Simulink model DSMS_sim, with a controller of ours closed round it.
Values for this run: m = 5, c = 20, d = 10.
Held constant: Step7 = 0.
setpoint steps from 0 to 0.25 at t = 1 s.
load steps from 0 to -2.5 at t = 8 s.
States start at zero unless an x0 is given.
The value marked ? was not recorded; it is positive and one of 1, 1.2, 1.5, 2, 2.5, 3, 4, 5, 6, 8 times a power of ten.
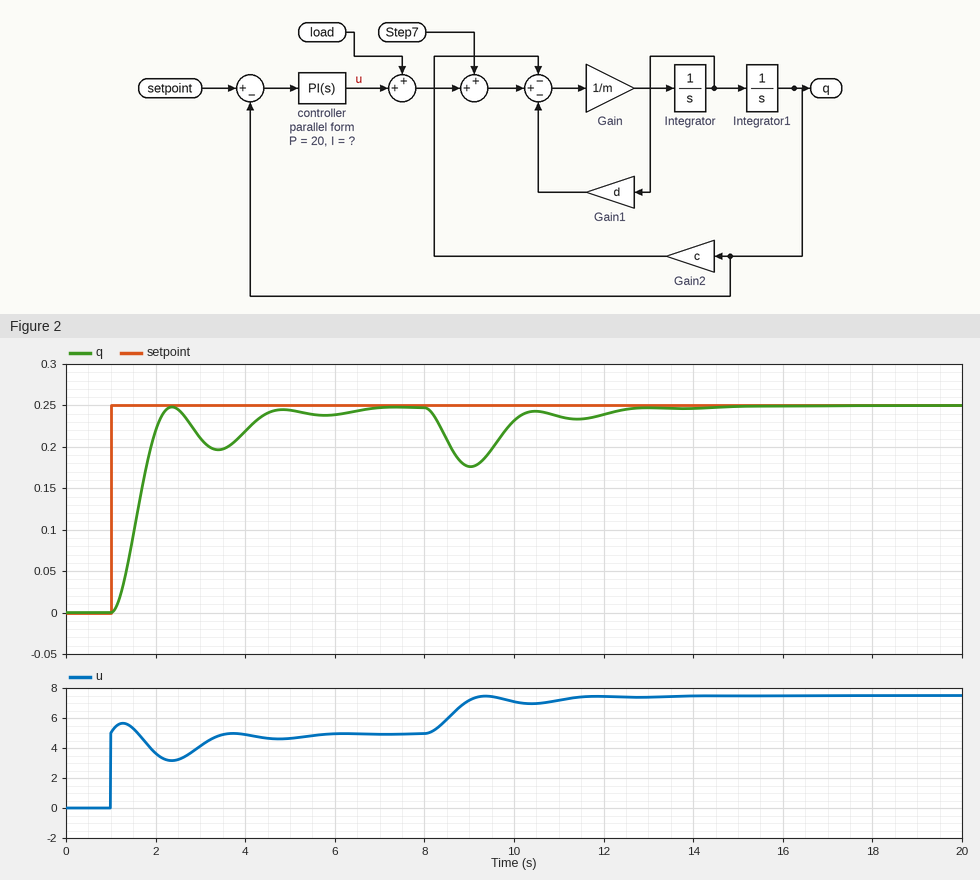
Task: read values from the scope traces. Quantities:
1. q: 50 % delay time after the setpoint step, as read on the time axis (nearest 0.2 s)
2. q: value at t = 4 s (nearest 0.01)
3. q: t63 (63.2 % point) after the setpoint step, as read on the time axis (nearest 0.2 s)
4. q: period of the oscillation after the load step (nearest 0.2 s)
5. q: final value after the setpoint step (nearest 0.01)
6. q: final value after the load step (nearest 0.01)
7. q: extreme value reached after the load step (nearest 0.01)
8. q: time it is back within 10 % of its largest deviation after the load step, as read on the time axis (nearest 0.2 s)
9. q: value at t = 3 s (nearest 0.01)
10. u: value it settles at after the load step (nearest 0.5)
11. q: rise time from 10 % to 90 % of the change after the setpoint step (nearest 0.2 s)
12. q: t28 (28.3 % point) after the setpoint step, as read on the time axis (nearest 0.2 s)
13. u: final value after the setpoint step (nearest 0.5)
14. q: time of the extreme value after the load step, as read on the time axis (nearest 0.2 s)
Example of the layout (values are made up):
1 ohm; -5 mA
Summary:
1.6 s; 0.22; 1.8 s; 2.4 s; 0.25; 0.25; 0.18; 12.2 s; 0.21; 7.5; 0.8 s; 1.4 s; 5.0; 9.0 s
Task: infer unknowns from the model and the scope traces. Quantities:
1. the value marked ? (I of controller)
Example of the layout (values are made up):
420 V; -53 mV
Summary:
20
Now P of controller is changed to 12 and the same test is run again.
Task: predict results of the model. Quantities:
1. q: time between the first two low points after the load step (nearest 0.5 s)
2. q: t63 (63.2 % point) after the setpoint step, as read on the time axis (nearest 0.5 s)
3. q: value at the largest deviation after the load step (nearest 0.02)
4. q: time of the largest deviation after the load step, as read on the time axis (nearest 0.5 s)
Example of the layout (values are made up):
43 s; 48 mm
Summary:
3.0 s; 2.0 s; 0.16; 9.0 s
